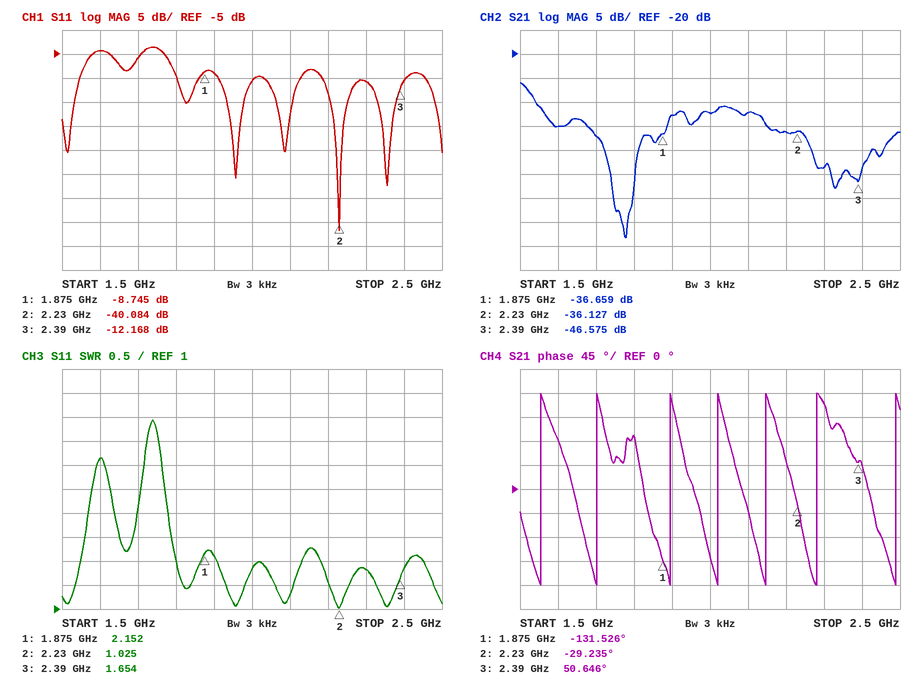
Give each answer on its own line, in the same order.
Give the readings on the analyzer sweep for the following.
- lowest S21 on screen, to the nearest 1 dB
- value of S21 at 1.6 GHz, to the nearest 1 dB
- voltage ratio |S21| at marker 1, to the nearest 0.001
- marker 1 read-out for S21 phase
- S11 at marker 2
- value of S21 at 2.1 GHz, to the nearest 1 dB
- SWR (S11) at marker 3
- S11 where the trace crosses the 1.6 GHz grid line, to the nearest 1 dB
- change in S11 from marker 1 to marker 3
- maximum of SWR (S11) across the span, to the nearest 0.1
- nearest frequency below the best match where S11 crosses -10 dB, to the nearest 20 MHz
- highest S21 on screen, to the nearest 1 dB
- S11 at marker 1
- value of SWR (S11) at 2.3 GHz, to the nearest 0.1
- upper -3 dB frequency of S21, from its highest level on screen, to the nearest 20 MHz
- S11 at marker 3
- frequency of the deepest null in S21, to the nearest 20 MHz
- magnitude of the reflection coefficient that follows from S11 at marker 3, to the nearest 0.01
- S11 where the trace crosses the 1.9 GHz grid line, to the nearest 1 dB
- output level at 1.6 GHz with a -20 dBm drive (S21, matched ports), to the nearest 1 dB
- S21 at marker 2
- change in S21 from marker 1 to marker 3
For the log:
-58 dB
-35 dB
0.015
-131.526°
-40.084 dB
-32 dB
1.654
-4 dB
-3.423 dB
4.9
2.18 GHz
-26 dB
-8.745 dB
1.8
1.54 GHz
-12.168 dB
1.78 GHz
0.25
-9 dB
-55 dBm
-36.127 dB
-9.916 dB
